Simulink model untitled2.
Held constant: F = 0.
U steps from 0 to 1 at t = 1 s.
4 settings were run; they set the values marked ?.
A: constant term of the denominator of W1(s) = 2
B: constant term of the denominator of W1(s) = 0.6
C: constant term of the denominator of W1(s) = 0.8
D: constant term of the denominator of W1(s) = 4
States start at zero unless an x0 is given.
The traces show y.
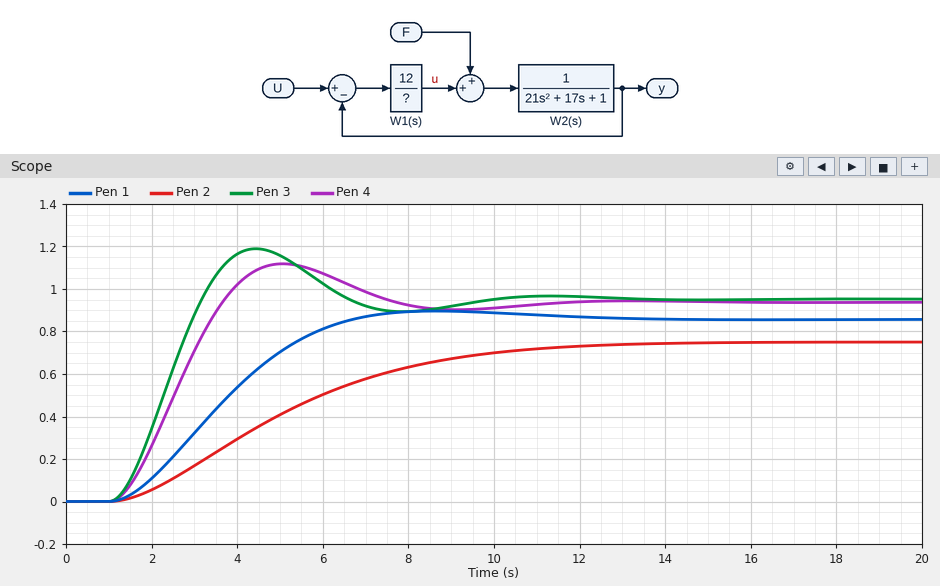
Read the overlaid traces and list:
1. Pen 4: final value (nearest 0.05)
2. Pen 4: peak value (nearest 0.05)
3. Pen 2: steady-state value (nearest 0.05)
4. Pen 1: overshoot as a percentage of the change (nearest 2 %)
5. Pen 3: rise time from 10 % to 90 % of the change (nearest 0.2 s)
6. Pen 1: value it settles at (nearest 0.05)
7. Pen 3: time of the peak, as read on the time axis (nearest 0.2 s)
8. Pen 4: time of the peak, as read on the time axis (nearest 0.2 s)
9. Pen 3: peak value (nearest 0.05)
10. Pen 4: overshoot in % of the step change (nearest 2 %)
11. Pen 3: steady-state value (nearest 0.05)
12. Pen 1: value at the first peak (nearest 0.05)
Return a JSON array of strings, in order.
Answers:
["0.95", "1.10", "0.75", "4 %", "1.4 s", "0.85", "4.4 s", "5.0 s", "1.20", "20 %", "0.95", "0.90"]
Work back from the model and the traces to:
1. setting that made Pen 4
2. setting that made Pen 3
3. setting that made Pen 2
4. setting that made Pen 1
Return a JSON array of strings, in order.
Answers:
["C", "B", "D", "A"]
